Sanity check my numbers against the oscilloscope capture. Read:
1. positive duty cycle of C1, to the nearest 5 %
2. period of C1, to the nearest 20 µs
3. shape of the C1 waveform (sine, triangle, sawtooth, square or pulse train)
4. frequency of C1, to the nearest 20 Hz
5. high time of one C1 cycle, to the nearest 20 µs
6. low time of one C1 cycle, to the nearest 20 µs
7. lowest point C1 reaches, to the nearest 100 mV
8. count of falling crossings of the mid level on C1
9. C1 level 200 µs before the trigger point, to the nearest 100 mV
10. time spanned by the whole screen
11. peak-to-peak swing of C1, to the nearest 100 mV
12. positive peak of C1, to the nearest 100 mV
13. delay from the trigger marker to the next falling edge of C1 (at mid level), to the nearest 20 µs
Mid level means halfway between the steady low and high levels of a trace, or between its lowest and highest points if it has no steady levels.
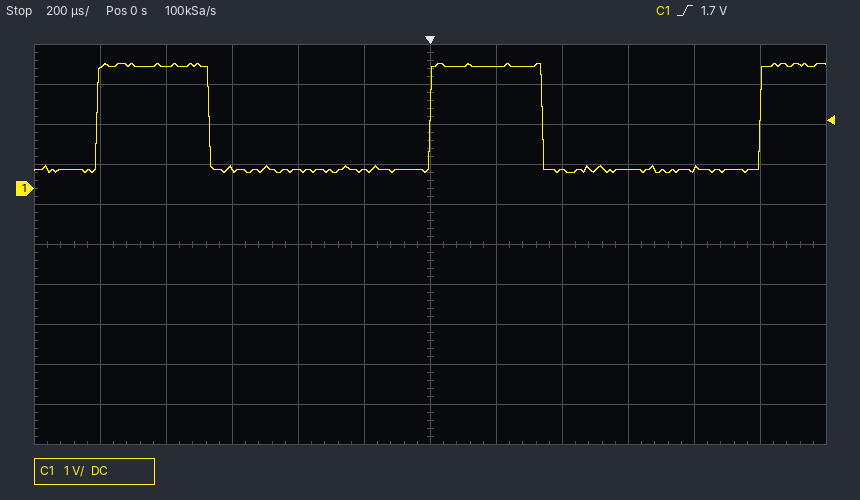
35 %
1.00 ms
pulse train
1.00 kHz
340 µs
660 µs
400 mV
2
500 mV
2.4 ms
2.7 V
3.1 V
340 µs
